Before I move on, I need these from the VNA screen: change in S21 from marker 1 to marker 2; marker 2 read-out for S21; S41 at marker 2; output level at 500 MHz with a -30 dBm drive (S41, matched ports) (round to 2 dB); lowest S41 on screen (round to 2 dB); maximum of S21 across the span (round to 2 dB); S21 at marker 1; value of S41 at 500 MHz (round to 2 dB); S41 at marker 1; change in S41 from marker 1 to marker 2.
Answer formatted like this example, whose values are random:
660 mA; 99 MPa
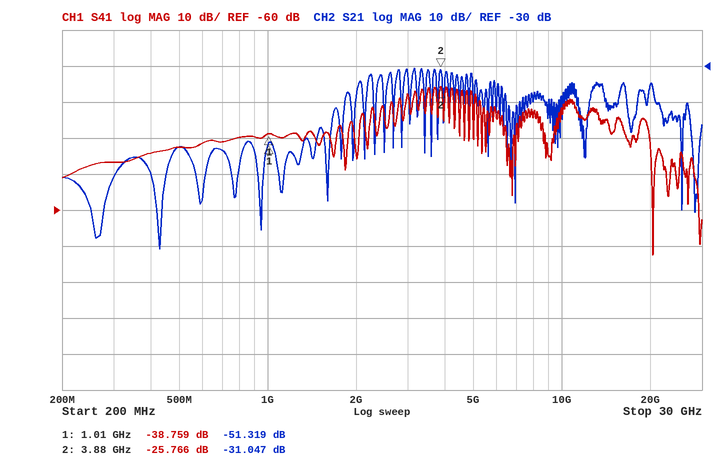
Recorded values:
20.272 dB; -31.047 dB; -25.766 dB; -72 dBm; -72 dB; -30 dB; -51.319 dB; -42 dB; -38.759 dB; 12.993 dB
